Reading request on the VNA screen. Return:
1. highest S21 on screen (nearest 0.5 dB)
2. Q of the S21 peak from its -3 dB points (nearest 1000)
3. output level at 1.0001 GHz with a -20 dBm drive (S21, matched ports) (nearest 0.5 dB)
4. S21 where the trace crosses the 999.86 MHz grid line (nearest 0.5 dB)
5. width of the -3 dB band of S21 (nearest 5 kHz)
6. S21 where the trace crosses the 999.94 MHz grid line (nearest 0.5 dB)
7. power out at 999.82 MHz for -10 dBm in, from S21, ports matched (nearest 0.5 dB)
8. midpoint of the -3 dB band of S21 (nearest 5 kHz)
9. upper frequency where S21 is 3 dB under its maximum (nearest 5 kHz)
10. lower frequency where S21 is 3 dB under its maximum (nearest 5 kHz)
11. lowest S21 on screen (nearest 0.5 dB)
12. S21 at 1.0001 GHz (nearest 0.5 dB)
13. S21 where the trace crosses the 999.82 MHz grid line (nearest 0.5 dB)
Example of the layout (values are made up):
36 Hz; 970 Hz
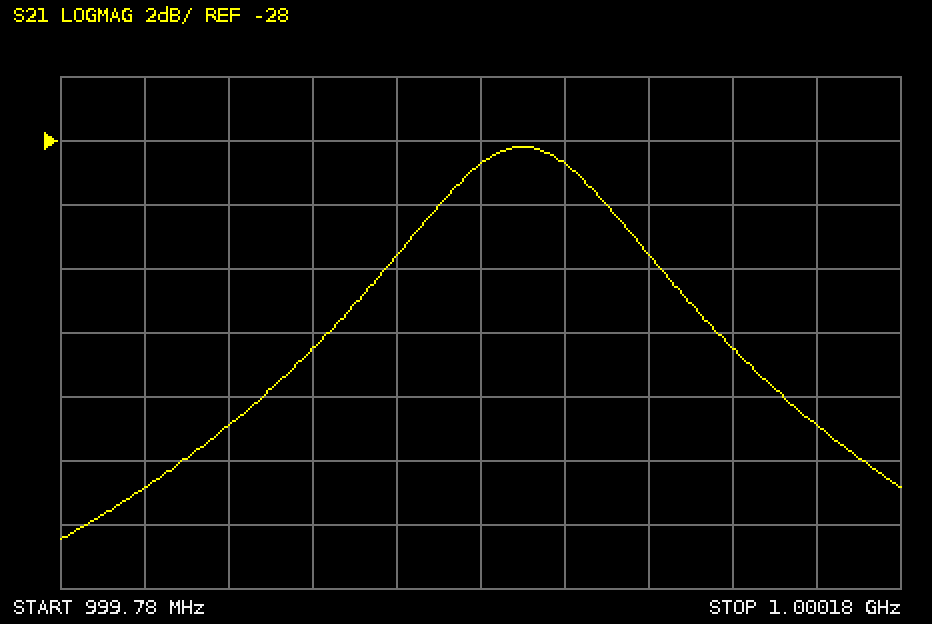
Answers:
-28.0 dB; 9000; -54.5 dBm; -37.0 dB; 110 kHz; -31.5 dB; -49.0 dBm; 1.000000 GHz; 1.000055 GHz; 999.945 MHz; -40.5 dB; -34.5 dB; -39.0 dB
